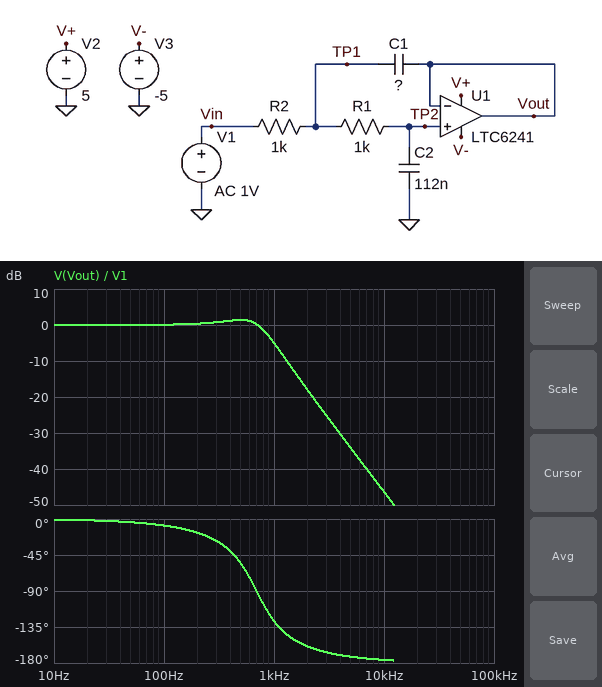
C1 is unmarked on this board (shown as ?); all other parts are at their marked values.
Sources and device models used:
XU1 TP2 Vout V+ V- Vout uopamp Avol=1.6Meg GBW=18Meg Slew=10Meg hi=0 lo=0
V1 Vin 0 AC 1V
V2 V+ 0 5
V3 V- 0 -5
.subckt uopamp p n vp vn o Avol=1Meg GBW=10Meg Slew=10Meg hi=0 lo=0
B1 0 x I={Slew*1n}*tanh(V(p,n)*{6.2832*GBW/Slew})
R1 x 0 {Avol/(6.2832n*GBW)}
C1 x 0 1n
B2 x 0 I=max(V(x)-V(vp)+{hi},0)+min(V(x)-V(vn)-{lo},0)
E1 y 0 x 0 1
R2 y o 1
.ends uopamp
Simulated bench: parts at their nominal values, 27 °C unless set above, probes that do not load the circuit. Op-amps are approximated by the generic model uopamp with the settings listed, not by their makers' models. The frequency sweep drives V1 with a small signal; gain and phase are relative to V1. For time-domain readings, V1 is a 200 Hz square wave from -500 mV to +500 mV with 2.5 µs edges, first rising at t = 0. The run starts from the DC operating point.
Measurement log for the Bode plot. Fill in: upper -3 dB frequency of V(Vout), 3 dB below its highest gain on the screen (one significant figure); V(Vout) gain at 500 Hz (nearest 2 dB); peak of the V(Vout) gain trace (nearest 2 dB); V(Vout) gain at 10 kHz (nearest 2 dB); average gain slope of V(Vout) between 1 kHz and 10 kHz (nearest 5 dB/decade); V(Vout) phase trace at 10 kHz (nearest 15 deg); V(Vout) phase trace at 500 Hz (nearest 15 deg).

800 Hz
2 dB
2 dB
-46 dB
-40 dB/decade
-180 deg
-60 deg
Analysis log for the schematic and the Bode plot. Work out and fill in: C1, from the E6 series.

470 nF
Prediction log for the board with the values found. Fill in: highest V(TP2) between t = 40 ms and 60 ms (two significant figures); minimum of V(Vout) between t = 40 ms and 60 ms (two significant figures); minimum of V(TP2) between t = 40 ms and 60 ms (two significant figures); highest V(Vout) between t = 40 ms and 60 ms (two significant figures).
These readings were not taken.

670 mV
-670 mV
-670 mV
670 mV
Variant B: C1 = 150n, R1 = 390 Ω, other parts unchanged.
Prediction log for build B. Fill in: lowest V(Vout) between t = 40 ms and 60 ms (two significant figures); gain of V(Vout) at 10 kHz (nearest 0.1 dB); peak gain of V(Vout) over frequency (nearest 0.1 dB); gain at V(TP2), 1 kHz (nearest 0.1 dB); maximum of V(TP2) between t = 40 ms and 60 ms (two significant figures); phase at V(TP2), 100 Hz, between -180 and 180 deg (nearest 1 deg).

-500 mV
-28.5 dB
0 dB
-1.8 dB
500 mV
-6 deg
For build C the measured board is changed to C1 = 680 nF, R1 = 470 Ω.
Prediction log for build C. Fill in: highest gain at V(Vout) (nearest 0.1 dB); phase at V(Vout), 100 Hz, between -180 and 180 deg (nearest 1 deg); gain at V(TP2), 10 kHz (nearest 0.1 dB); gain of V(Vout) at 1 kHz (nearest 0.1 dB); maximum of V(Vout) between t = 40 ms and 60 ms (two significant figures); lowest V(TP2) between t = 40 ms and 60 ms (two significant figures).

2.1 dB
-6 deg
-43.0 dB
-0.9 dB
720 mV
-720 mV
